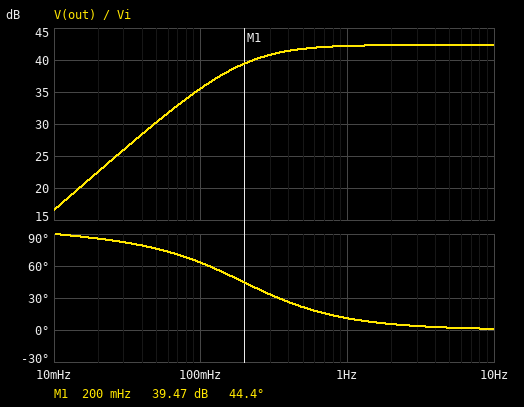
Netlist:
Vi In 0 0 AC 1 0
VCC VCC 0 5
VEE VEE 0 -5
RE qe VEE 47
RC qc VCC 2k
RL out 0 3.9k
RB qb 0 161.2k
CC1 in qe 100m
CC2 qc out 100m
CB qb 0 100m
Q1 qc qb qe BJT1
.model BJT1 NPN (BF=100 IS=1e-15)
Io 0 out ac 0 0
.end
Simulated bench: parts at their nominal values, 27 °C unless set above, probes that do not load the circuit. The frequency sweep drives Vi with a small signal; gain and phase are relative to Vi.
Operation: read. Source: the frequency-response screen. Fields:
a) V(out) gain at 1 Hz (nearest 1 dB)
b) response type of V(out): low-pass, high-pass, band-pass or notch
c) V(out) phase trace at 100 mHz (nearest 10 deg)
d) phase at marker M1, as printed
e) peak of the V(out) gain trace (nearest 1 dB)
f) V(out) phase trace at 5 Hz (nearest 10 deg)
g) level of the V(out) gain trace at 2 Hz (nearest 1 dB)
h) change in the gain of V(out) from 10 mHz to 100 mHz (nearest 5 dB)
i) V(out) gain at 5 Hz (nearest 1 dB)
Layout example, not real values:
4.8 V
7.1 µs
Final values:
42 dB
high-pass
60 deg
44.4 deg
42 dB
0 deg
42 dB
20 dB
42 dB
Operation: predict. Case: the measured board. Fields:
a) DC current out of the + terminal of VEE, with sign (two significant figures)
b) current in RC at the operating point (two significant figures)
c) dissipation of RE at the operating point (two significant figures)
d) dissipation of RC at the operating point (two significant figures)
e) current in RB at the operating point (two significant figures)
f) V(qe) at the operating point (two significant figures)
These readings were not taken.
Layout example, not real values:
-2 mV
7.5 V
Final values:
-2.6 mA
2.6 mA
320 µW
13 mW
26 µA
-4.9 V
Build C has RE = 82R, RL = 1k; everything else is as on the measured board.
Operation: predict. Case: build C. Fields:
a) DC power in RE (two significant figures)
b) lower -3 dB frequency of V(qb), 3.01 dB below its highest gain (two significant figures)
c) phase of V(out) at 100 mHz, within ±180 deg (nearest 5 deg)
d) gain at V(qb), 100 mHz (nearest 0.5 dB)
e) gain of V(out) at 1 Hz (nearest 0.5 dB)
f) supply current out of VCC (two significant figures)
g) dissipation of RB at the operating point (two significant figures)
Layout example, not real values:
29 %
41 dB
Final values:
530 µW
180 µHz
60 deg
-42.5 dB
36.0 dB
2.5 mA
100 µW
